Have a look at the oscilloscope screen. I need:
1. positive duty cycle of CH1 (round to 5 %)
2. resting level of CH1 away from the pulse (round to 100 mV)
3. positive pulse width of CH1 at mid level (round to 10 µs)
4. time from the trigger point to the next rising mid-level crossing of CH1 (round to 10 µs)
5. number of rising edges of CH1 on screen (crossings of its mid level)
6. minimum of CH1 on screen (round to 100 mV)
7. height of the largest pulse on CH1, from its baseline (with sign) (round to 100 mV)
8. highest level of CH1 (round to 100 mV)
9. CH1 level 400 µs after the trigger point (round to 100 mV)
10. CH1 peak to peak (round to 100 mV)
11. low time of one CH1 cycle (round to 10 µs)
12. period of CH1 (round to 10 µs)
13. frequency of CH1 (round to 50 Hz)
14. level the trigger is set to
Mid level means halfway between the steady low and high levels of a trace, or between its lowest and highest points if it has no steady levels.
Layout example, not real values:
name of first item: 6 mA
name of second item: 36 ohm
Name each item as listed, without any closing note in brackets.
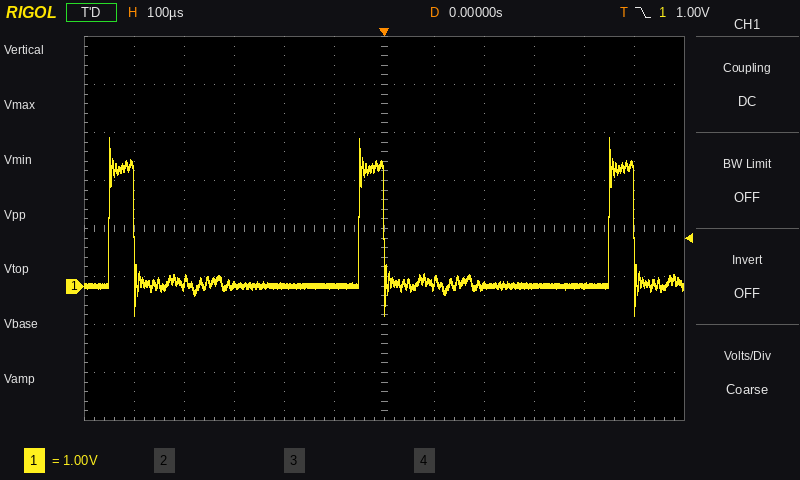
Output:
positive duty cycle of CH1: 10 %
resting level of CH1 away from the pulse: 0.0 V
positive pulse width of CH1 at mid level: 50 µs
time from the trigger point to the next rising mid-level crossing of CH1: 450 µs
number of rising edges of CH1 on screen: 3
minimum of CH1 on screen: -600 mV
height of the largest pulse on CH1, from its baseline (with sign): +3.1 V
highest level of CH1: 3.1 V
CH1 level 400 µs after the trigger point: 0.0 V
CH1 peak to peak: 3.7 V
low time of one CH1 cycle: 450 µs
period of CH1: 500 µs
frequency of CH1: 2.00 kHz
level the trigger is set to: 1.00 V
